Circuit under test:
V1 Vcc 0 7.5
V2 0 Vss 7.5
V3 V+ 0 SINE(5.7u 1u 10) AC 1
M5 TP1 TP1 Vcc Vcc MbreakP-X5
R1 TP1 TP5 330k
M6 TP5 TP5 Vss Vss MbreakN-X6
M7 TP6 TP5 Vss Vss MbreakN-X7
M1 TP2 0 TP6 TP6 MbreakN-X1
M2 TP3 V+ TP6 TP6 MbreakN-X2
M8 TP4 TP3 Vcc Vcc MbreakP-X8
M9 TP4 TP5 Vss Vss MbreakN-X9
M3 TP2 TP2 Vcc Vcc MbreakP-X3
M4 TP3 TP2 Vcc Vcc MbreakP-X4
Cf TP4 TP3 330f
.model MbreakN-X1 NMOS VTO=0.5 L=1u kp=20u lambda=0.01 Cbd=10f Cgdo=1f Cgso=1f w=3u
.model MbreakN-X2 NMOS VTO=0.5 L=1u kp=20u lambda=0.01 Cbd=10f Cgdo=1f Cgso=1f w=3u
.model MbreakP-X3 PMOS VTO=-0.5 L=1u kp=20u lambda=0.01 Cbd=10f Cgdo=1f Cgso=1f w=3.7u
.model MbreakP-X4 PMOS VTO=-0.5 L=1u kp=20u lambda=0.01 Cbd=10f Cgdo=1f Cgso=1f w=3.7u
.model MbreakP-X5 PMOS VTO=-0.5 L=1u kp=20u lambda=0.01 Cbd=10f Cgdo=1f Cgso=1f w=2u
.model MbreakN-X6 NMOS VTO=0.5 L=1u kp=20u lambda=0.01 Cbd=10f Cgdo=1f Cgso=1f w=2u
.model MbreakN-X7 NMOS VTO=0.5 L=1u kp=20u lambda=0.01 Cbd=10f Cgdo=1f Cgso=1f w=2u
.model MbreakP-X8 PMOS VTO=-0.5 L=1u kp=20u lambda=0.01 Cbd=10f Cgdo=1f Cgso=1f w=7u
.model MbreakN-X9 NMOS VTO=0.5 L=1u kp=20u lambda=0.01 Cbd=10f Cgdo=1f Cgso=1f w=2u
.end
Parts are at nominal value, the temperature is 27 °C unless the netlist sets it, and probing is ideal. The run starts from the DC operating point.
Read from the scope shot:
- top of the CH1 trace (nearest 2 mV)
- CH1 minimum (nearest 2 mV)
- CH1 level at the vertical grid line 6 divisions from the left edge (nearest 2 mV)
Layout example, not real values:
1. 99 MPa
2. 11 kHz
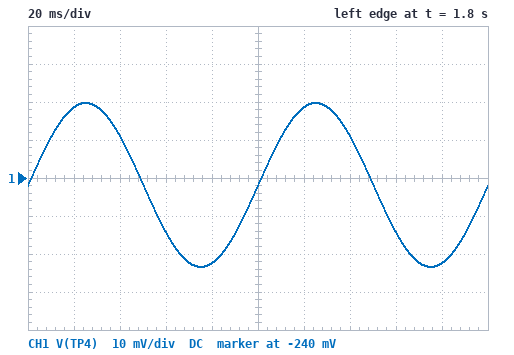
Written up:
1. -220 mV
2. -264 mV
3. -222 mV
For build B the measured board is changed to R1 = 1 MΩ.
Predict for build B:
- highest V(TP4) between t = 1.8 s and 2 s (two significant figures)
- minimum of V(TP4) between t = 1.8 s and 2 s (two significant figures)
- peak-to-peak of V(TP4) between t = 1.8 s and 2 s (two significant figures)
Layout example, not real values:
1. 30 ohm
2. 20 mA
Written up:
1. 330 mV
2. 210 mV
3. 120 mV
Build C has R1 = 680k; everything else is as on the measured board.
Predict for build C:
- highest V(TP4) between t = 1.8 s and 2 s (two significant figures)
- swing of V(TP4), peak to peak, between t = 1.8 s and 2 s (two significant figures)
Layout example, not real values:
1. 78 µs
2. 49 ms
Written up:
1. 120 mV
2. 83 mV
